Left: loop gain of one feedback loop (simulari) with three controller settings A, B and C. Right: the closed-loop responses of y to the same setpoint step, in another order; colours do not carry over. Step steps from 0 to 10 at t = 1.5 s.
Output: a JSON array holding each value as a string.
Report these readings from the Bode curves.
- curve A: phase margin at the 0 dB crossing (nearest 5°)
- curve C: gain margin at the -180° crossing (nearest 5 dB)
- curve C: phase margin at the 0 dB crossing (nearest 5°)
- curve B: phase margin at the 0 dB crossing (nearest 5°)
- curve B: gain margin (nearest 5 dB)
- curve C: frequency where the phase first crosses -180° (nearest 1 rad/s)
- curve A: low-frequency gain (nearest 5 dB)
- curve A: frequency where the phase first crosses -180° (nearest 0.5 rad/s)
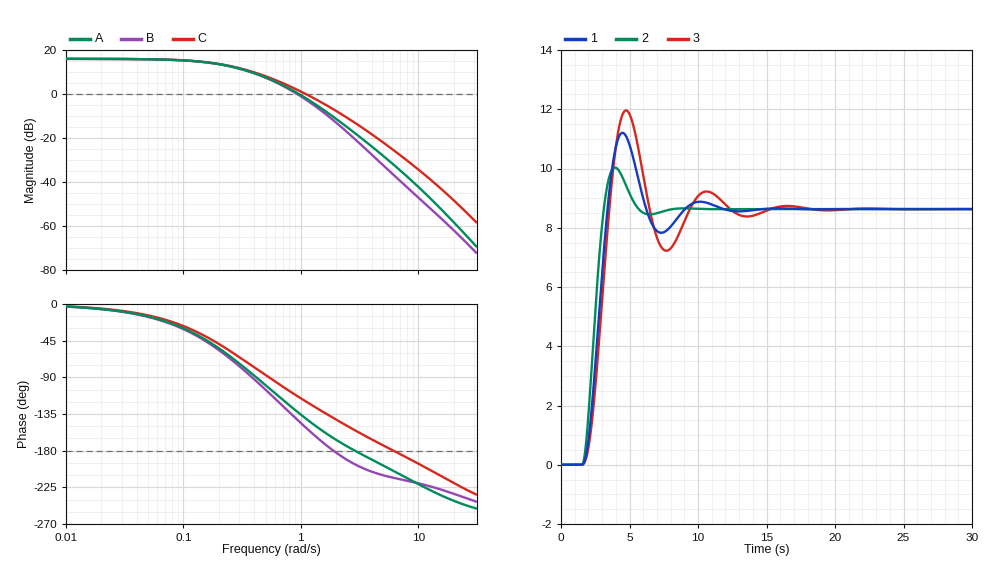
["45°", "25 dB", "60°", "40°", "10 dB", "6 rad/s", "15 dB", "3.0 rad/s"]
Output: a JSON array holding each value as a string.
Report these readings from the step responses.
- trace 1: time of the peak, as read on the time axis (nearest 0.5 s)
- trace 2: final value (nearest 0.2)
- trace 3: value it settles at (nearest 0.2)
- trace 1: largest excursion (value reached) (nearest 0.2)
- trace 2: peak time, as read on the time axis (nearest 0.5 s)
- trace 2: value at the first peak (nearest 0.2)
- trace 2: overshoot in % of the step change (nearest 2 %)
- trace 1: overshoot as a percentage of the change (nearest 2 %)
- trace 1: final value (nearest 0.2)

["4.5 s", "8.6", "8.6", "11.2", "4.0 s", "10.0", "16 %", "30 %", "8.6"]
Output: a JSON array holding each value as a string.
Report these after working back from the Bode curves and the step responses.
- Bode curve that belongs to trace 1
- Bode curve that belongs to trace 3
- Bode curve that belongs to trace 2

["A", "B", "C"]
